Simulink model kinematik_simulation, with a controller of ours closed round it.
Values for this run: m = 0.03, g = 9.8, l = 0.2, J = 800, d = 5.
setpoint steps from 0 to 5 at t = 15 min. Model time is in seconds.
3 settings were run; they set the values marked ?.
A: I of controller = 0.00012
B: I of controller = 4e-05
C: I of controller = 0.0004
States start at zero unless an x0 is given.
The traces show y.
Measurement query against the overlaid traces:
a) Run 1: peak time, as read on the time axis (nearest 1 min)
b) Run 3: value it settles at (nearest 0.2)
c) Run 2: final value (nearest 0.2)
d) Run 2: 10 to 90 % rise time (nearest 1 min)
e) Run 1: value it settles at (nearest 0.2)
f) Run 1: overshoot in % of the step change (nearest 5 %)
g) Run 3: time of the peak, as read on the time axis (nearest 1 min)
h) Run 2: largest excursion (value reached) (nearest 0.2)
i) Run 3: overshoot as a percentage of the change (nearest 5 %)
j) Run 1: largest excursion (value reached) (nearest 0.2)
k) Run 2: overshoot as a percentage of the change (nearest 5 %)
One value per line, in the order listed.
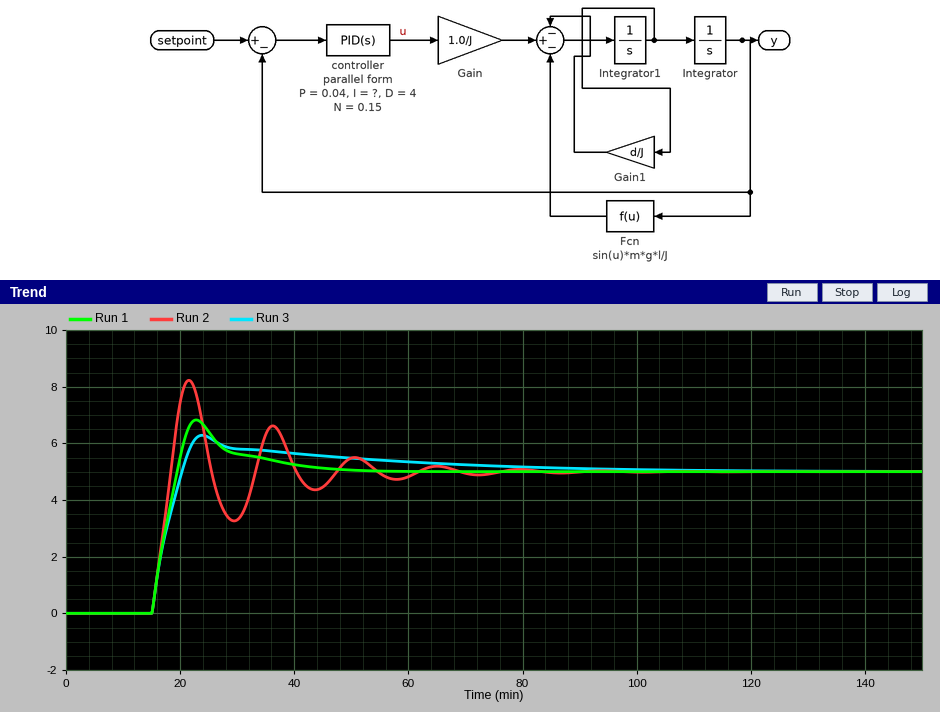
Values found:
23 min
5.0
5.0
3 min
5.0
35 %
24 min
8.2
25 %
6.8
65 %
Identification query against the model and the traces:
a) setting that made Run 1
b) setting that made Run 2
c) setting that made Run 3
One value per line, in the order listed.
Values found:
A
C
B
